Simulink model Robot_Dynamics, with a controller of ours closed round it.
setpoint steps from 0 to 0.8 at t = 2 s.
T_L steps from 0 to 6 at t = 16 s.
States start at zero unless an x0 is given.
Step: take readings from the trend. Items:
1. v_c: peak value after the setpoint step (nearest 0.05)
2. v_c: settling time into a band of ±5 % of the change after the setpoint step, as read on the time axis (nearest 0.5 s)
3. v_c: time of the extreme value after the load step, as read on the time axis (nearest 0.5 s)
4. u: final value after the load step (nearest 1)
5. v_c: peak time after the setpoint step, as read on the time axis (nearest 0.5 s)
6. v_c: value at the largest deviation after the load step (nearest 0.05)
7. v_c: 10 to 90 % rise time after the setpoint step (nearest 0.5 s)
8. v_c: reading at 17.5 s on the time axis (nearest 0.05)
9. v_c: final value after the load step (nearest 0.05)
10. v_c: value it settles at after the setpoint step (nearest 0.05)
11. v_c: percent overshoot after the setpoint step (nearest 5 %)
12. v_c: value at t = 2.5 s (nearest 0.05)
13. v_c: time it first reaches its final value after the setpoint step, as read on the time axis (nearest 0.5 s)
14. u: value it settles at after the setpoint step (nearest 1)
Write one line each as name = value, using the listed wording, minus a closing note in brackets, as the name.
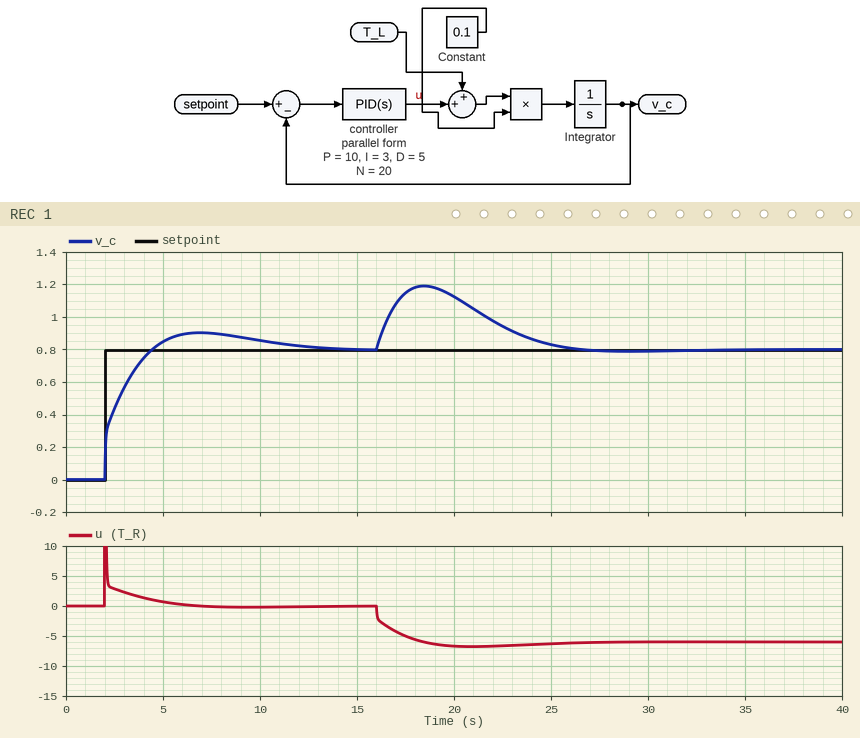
v_c: peak value after the setpoint step = 0.90
v_c: settling time into a band of ±5 % of the change after the setpoint step, as read on the time axis = 11.0 s
v_c: time of the extreme value after the load step, as read on the time axis = 18.5 s
u: final value after the load step = -6
v_c: peak time after the setpoint step, as read on the time axis = 7.0 s
v_c: value at the largest deviation after the load step = 1.20
v_c: 10 to 90 % rise time after the setpoint step = 2.0 s
v_c: reading at 17.5 s on the time axis = 1.15
v_c: final value after the load step = 0.80
v_c: value it settles at after the setpoint step = 0.80
v_c: percent overshoot after the setpoint step = 15 %
v_c: value at t = 2.5 s = 0.45
v_c: time it first reaches its final value after the setpoint step, as read on the time axis = 4.5 s
u: value it settles at after the setpoint step = 0
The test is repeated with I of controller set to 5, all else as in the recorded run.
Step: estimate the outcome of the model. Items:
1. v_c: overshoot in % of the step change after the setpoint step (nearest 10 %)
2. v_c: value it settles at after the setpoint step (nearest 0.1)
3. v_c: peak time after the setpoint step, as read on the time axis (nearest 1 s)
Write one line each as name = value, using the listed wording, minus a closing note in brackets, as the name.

v_c: overshoot in % of the step change after the setpoint step = 20 %
v_c: value it settles at after the setpoint step = 0.8
v_c: peak time after the setpoint step, as read on the time axis = 6 s
